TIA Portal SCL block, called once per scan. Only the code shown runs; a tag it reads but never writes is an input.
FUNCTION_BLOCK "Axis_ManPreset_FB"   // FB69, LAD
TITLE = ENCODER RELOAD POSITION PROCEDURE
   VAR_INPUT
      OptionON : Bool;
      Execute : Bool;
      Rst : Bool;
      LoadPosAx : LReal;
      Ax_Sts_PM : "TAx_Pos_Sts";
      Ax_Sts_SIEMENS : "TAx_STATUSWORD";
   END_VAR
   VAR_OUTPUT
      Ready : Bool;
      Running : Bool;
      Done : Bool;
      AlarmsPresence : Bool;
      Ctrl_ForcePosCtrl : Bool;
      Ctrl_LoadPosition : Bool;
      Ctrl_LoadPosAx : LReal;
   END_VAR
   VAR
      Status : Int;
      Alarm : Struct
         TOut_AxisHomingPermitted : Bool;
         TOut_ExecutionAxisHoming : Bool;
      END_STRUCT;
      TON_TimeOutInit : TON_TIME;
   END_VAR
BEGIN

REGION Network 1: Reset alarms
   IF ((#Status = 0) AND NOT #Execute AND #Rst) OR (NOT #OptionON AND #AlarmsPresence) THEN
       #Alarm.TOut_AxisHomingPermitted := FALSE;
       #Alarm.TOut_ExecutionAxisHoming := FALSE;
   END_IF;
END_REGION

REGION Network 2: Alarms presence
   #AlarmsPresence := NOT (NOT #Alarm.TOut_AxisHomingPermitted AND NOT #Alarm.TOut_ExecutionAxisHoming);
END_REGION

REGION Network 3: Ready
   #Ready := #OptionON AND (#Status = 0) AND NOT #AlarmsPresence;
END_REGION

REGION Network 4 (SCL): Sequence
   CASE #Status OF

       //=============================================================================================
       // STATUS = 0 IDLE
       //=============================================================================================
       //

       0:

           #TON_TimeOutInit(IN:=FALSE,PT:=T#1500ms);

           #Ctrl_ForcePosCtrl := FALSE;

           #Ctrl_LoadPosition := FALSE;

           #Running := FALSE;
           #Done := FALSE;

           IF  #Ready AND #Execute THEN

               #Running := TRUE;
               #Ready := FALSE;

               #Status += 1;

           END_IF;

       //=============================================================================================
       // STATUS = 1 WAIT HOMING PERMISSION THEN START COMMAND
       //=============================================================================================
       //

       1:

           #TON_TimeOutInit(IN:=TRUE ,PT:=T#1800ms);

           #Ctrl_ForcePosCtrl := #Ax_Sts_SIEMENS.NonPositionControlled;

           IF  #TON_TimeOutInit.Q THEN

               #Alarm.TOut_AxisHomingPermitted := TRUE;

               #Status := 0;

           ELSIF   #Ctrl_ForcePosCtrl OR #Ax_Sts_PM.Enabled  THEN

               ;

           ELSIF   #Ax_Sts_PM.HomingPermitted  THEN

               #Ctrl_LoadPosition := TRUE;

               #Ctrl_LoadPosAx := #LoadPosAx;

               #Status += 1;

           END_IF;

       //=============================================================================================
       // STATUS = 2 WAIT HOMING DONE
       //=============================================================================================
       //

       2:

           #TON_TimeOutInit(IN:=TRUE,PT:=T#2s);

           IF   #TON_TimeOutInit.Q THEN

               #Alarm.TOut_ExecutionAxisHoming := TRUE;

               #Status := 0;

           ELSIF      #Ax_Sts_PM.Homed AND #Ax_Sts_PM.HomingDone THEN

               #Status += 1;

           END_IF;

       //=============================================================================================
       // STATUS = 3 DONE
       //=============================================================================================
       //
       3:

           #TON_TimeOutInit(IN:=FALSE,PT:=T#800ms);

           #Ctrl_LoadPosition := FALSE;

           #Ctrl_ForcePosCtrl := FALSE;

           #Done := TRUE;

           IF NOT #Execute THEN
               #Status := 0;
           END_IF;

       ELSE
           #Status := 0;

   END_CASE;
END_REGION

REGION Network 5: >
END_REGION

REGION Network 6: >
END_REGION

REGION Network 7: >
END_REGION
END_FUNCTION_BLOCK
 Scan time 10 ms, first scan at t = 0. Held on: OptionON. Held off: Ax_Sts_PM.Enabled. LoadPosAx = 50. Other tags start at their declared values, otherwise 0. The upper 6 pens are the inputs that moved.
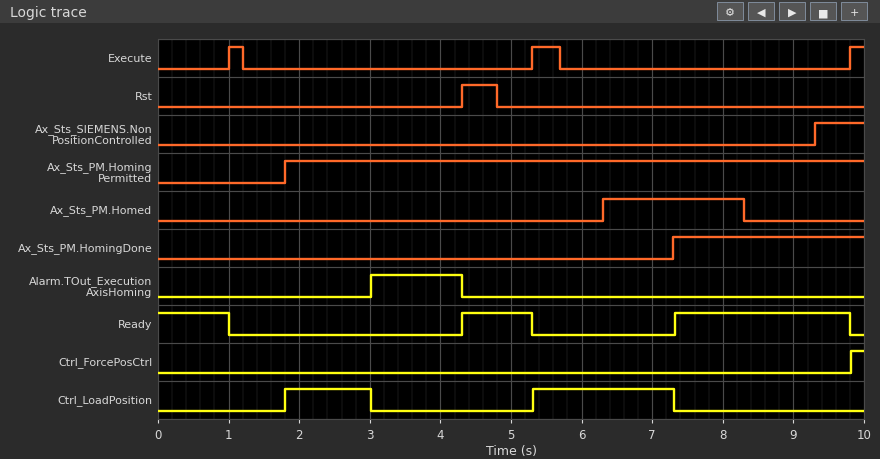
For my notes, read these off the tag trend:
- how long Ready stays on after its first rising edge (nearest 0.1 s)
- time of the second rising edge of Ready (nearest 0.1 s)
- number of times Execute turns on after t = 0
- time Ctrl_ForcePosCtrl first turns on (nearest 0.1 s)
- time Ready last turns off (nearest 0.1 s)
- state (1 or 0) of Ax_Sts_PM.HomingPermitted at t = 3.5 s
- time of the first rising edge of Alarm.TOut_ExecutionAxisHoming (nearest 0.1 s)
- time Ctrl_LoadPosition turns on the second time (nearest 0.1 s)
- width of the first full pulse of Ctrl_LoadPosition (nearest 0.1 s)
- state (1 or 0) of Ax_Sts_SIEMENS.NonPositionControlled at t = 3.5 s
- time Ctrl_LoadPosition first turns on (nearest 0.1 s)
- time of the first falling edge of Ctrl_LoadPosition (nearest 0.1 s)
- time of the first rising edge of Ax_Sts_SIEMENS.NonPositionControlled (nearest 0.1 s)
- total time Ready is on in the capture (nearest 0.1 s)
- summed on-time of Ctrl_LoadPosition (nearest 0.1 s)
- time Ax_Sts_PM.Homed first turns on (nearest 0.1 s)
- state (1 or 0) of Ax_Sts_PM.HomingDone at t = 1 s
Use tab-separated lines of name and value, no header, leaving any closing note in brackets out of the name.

how long Ready stays on after its first rising edge	1.0 s
time of the second rising edge of Ready	7.3 s
number of times Execute turns on after t = 0	3
time Ctrl_ForcePosCtrl first turns on	9.8 s
time Ready last turns off	9.8 s
state (1 or 0) of Ax_Sts_PM.HomingPermitted at t = 3.5 s	1
time of the first rising edge of Alarm.TOut_ExecutionAxisHoming	3.0 s
time Ctrl_LoadPosition turns on the second time	5.3 s
width of the first full pulse of Ctrl_LoadPosition	1.2 s
state (1 or 0) of Ax_Sts_SIEMENS.NonPositionControlled at t = 3.5 s	0
time Ctrl_LoadPosition first turns on	1.8 s
time of the first falling edge of Ctrl_LoadPosition	3.0 s
time of the first rising edge of Ax_Sts_SIEMENS.NonPositionControlled	9.3 s
total time Ready is on in the capture	4.5 s
summed on-time of Ctrl_LoadPosition	3.2 s
time Ax_Sts_PM.Homed first turns on	6.3 s
state (1 or 0) of Ax_Sts_PM.HomingDone at t = 1 s	0
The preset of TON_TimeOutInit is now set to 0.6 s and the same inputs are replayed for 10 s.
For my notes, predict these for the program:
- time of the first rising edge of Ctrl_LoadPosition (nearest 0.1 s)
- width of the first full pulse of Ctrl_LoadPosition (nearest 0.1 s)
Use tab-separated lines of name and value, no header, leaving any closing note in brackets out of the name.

time of the first rising edge of Ctrl_LoadPosition	5.3 s
width of the first full pulse of Ctrl_LoadPosition	2.0 s
